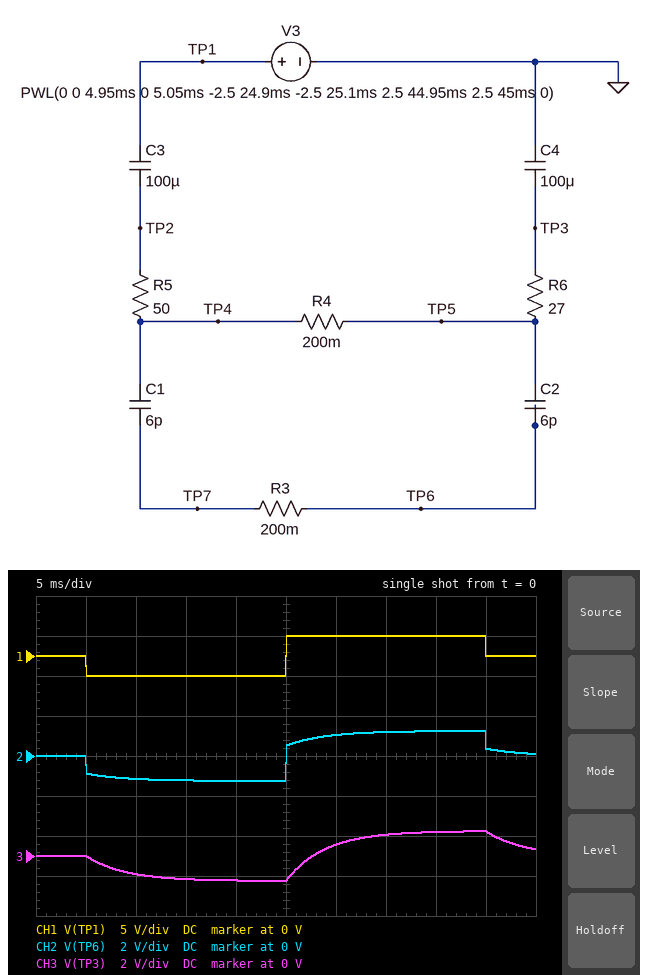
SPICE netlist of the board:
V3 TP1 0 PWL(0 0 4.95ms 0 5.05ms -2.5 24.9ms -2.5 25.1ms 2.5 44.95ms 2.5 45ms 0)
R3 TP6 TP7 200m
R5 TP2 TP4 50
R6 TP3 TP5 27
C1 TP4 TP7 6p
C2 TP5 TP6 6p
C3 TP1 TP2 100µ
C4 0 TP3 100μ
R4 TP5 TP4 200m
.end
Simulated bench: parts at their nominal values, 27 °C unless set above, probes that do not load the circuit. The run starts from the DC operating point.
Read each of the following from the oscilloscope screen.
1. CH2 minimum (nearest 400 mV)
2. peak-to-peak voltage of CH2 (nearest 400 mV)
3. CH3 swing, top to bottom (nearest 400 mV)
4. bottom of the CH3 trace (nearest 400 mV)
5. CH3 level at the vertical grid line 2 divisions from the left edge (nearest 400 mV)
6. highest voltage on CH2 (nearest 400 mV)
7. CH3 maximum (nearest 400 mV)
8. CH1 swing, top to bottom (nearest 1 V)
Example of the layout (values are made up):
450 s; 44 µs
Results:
-1.2 V; 2.4 V; 2.4 V; -1.2 V; -800 mV; 1.2 V; 1.2 V; 5 V
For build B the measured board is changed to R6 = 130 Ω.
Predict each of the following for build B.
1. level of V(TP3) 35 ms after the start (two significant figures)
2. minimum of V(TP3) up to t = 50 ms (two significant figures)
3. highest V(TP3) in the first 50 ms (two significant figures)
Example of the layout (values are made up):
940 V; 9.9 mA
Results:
470 mV; -1.1 V; 990 mV
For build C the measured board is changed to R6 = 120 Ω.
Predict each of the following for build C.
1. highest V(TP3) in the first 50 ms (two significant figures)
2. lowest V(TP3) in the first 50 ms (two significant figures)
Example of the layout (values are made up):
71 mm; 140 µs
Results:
1.0 V; -1.1 V
